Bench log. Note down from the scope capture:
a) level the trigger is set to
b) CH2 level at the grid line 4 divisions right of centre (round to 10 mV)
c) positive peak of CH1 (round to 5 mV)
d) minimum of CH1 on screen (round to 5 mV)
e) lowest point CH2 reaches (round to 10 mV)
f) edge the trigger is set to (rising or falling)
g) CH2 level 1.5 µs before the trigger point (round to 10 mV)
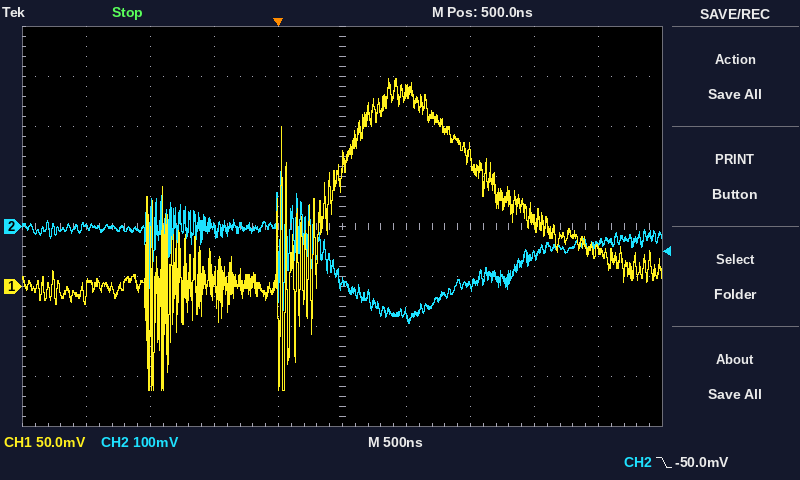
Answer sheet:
-50.0 mV
-30 mV
210 mV
-105 mV
-190 mV
falling
0 mV
